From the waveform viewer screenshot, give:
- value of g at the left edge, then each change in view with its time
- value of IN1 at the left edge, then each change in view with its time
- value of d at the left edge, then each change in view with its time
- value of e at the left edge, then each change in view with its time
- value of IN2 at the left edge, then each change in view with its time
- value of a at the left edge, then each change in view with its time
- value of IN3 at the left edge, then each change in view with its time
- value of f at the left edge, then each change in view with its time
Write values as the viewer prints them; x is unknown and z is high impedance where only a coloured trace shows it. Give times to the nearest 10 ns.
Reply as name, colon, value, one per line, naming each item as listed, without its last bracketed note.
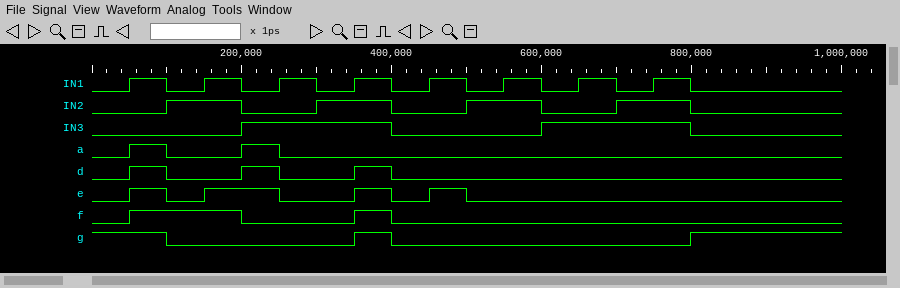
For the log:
value of g at the left edge, then each change in view with its time: 1, 0 at 100 ns, 1 at 350 ns, 0 at 400 ns, 1 at 800 ns
value of IN1 at the left edge, then each change in view with its time: 0, 1 at 50 ns, 0 at 100 ns, 1 at 150 ns, 0 at 200 ns, 1 at 250 ns, 0 at 300 ns, 1 at 350 ns, 0 at 400 ns, 1 at 450 ns, 0 at 500 ns, 1 at 550 ns, 0 at 600 ns, 1 at 650 ns, 0 at 700 ns, 1 at 750 ns, 0 at 800 ns
value of d at the left edge, then each change in view with its time: 0, 1 at 50 ns, 0 at 100 ns, 1 at 200 ns, 0 at 250 ns, 1 at 350 ns, 0 at 400 ns
value of e at the left edge, then each change in view with its time: 0, 1 at 50 ns, 0 at 100 ns, 1 at 150 ns, 0 at 250 ns, 1 at 350 ns, 0 at 400 ns, 1 at 450 ns, 0 at 500 ns
value of IN2 at the left edge, then each change in view with its time: 0, 1 at 100 ns, 0 at 200 ns, 1 at 300 ns, 0 at 400 ns, 1 at 500 ns, 0 at 600 ns, 1 at 700 ns, 0 at 800 ns
value of a at the left edge, then each change in view with its time: 0, 1 at 50 ns, 0 at 100 ns, 1 at 200 ns, 0 at 250 ns
value of IN3 at the left edge, then each change in view with its time: 0, 1 at 200 ns, 0 at 400 ns, 1 at 600 ns, 0 at 800 ns
value of f at the left edge, then each change in view with its time: 0, 1 at 50 ns, 0 at 200 ns, 1 at 350 ns, 0 at 400 ns
